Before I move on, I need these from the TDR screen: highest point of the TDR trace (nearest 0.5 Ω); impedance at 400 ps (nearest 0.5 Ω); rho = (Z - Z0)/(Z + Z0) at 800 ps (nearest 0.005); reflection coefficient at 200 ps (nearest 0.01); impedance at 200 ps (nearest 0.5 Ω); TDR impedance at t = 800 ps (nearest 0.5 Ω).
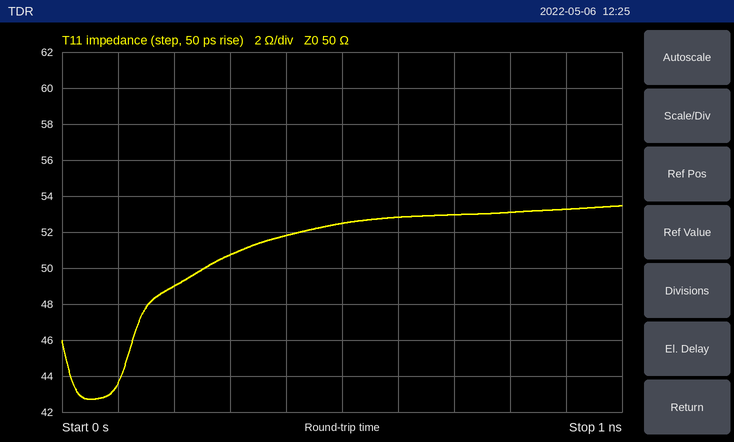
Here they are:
53.5 Ω
52.0 Ω
+0.030
-0.01
49.0 Ω
53.0 Ω
